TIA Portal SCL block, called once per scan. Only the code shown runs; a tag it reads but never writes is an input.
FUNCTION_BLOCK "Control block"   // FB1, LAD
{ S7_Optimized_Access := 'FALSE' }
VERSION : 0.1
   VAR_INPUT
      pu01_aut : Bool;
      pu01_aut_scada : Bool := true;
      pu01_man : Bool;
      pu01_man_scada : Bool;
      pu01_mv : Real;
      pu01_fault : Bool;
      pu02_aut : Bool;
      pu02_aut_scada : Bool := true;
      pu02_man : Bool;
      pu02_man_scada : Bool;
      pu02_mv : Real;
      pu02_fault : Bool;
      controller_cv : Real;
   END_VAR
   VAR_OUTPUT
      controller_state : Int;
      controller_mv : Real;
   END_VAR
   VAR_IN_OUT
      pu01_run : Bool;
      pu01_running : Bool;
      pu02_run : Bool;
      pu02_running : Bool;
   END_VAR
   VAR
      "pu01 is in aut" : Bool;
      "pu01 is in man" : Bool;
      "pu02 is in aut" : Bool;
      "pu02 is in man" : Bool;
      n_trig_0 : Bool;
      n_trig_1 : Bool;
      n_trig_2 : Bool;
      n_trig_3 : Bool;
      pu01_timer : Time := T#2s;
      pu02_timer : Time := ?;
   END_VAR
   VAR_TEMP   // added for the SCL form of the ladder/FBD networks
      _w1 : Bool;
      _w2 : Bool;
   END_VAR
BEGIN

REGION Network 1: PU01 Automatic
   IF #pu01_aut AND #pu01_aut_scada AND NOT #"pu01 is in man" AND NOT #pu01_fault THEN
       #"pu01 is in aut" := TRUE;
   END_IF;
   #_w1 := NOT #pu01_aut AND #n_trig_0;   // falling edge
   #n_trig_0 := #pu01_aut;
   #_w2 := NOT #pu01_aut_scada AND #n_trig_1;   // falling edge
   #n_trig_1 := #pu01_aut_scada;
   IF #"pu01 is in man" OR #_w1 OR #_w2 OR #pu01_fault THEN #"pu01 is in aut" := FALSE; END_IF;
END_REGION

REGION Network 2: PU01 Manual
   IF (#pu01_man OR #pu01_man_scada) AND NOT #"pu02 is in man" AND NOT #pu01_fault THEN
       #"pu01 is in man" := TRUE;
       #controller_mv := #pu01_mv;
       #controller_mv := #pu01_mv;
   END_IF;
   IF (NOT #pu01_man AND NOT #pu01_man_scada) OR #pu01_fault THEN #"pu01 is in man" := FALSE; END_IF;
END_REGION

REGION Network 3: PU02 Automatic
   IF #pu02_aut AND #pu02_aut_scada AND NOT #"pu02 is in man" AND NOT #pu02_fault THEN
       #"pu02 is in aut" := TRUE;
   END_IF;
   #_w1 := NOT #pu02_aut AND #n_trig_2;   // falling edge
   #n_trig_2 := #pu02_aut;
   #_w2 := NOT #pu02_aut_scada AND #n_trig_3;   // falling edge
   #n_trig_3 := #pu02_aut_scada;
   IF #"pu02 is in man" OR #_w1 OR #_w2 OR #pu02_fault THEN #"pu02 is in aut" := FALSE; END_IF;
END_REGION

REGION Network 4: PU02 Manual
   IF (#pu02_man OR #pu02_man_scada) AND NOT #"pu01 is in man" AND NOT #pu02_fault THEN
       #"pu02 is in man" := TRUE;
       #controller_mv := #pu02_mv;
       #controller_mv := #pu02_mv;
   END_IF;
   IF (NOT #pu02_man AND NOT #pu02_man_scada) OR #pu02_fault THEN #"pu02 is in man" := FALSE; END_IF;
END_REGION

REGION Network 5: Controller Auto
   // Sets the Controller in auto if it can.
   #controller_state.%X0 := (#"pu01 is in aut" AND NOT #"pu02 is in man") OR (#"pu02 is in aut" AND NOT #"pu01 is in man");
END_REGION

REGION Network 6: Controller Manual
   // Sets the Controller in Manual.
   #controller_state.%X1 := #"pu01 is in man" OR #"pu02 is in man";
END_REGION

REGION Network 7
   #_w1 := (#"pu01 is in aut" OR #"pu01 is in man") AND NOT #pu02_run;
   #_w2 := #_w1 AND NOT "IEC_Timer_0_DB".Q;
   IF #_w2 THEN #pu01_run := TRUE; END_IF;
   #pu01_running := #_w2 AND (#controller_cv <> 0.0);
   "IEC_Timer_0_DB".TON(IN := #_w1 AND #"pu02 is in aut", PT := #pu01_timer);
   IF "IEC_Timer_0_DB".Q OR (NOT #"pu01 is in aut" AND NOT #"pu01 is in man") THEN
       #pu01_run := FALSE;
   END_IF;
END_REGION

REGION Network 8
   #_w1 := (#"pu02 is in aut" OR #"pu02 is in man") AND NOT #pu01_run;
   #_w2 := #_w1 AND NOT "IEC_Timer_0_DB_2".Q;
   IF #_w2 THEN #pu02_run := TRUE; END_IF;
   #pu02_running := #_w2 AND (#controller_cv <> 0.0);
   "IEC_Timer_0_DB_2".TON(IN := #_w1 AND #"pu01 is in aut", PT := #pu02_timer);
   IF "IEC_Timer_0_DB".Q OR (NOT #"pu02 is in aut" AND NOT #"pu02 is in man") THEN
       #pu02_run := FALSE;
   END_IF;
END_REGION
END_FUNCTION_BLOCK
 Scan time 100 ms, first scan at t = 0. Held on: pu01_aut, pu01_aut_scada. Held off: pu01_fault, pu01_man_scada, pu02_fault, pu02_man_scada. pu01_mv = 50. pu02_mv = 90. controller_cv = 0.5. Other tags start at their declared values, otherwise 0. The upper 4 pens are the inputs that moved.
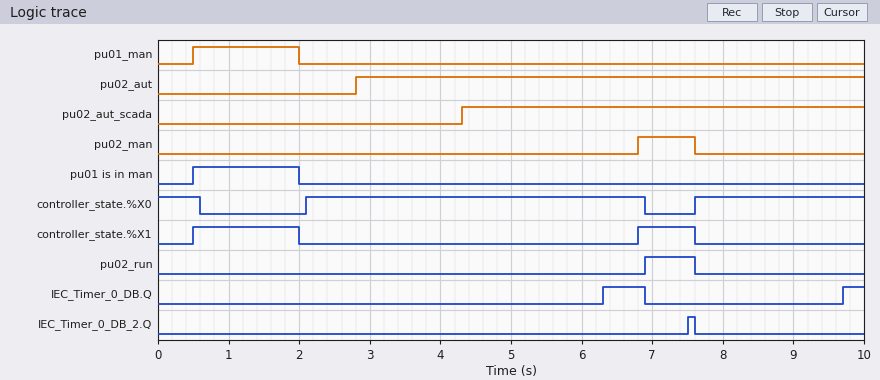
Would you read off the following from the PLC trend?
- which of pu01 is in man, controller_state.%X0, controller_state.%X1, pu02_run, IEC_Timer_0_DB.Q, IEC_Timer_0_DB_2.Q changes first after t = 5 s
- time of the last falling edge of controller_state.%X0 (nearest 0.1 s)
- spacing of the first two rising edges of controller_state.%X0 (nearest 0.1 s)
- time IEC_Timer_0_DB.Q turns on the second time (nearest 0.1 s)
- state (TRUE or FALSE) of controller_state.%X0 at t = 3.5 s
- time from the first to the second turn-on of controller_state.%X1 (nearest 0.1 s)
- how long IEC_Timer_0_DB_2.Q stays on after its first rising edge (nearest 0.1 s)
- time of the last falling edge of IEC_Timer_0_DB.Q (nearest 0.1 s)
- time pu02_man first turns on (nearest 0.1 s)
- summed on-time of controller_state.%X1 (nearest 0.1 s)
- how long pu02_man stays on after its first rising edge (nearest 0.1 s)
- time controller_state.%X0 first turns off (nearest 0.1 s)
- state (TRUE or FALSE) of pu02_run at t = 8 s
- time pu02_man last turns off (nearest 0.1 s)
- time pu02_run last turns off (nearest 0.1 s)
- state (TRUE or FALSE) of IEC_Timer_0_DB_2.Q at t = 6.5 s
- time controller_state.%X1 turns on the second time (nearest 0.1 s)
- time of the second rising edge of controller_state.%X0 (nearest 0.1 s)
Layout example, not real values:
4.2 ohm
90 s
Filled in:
IEC_Timer_0_DB.Q
6.9 s
5.5 s
9.7 s
TRUE
6.3 s
0.1 s
6.9 s
6.8 s
2.3 s
0.8 s
0.6 s
FALSE
7.6 s
7.6 s
FALSE
6.8 s
7.6 s
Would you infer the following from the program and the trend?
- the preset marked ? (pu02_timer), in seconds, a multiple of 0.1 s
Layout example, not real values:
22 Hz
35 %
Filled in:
1.2 s
